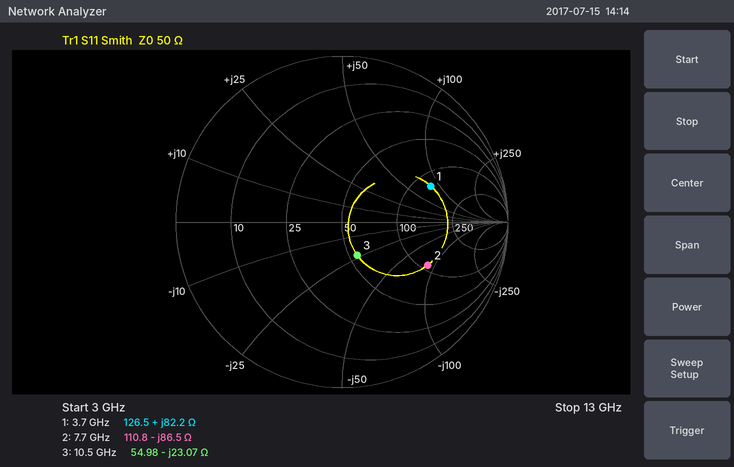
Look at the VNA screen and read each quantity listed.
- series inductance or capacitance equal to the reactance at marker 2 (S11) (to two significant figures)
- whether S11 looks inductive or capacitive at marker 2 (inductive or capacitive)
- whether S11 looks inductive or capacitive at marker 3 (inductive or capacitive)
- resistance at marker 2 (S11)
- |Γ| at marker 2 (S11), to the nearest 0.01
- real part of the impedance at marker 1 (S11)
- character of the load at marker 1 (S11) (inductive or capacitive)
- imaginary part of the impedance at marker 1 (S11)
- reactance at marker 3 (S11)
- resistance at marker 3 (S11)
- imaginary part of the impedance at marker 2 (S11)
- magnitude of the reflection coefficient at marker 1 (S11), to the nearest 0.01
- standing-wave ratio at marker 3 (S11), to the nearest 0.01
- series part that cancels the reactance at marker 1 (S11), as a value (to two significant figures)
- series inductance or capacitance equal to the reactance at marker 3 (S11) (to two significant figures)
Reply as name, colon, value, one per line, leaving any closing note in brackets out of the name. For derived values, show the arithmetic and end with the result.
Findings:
series inductance or capacitance equal to the reactance at marker 2 (S11): C = 1/(2π × 7.7 GHz × 86.5 Ω) ≈ 239 fF, so 240 fF to two significant figures
whether S11 looks inductive or capacitive at marker 2: capacitive
whether S11 looks inductive or capacitive at marker 3: capacitive
resistance at marker 2: 110.8 Ω
|Γ| at marker 2 (S11), to the nearest 0.01: 0.58
real part of the impedance at marker 1: 126.5 Ω
character of the load at marker 1 (S11): inductive
imaginary part of the impedance at marker 1: +82.2 Ω
reactance at marker 3: -23.07 Ω
resistance at marker 3: 54.98 Ω
imaginary part of the impedance at marker 2: -86.5 Ω
magnitude of the reflection coefficient at marker 1 (S11), to the nearest 0.01: 0.58
standing-wave ratio at marker 3 (S11), to the nearest 0.01: 1.56
series part that cancels the reactance at marker 1 (S11), as a value: C = 1/(2π × 3.7 GHz × 82.2 Ω) ≈ 523 fF, so 520 fF to two significant figures
series inductance or capacitance equal to the reactance at marker 3 (S11): C = 1/(2π × 10.5 GHz × 23.07 Ω) ≈ 657 fF, so 660 fF to two significant figures
